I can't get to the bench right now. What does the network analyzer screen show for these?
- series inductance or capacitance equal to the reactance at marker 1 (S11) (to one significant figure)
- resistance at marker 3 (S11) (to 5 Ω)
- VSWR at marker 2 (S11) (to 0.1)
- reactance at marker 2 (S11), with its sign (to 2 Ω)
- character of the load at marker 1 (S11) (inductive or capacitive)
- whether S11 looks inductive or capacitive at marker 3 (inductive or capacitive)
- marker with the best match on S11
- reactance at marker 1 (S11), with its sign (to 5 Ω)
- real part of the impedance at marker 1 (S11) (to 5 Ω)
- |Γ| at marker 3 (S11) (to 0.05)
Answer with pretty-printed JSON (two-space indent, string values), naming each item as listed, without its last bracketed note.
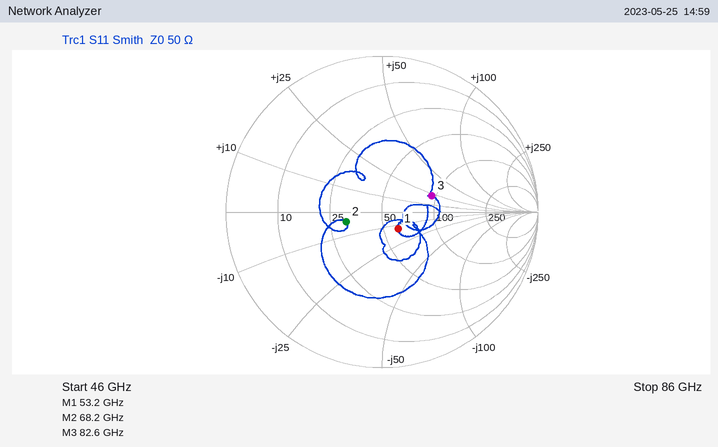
{
  "series inductance or capacitance equal to the reactance at marker 1 (S11)": "200 fF",
  "resistance at marker 3 (S11)": "95 Ω",
  "VSWR at marker 2 (S11)": "1.6",
  "reactance at marker 2 (S11), with its sign": "-4 Ω",
  "character of the load at marker 1 (S11)": "capacitive",
  "whether S11 looks inductive or capacitive at marker 3": "inductive",
  "marker with the best match on S11": "marker 1",
  "reactance at marker 1 (S11), with its sign": "-15 Ω",
  "real part of the impedance at marker 1 (S11)": "60 Ω",
  "|Γ| at marker 3 (S11)": "0.35"
}
